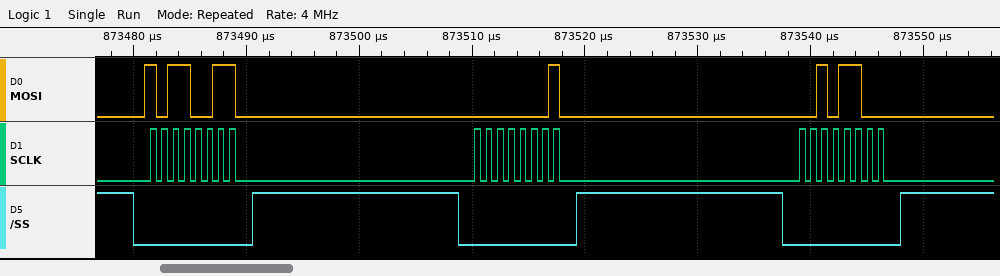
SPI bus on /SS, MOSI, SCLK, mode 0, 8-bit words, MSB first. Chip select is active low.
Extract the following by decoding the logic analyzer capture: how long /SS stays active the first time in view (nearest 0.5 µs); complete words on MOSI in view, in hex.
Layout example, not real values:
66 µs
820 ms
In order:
10.5 µs
B3, 01, 2C
